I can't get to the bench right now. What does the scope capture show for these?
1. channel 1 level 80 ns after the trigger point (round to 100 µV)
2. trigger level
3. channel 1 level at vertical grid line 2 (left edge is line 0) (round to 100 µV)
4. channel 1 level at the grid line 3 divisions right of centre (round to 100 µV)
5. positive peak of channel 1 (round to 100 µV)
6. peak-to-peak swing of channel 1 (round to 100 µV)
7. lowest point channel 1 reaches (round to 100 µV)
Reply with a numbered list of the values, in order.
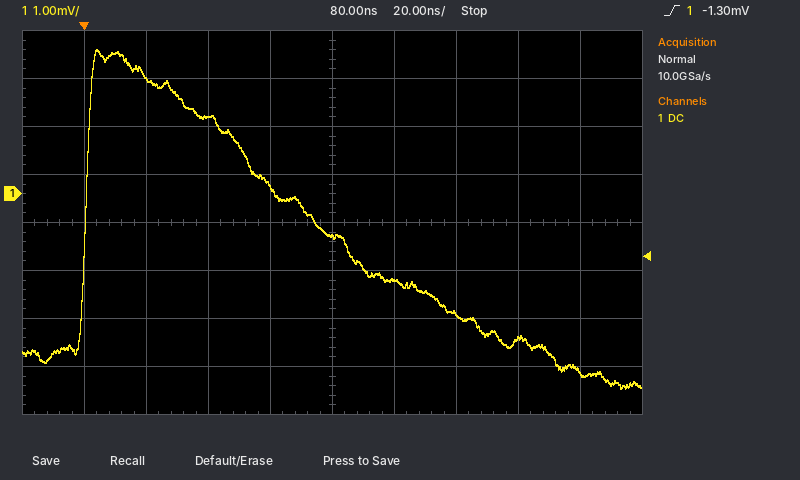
1. -900 µV
2. -1.30 mV
3. 2.4 mV
4. -3.0 mV
5. 3.0 mV
6. 7.1 mV
7. -4.1 mV
